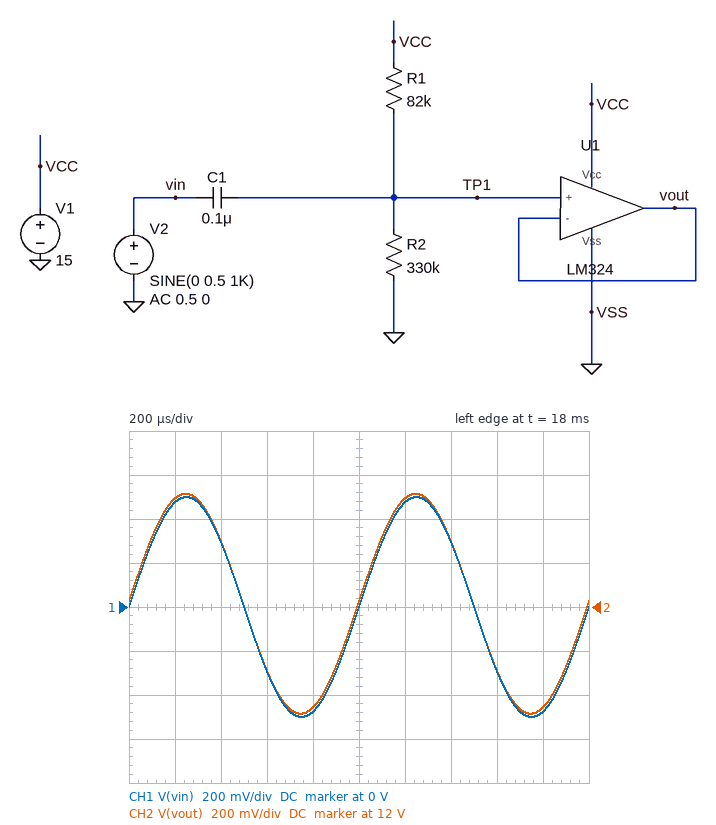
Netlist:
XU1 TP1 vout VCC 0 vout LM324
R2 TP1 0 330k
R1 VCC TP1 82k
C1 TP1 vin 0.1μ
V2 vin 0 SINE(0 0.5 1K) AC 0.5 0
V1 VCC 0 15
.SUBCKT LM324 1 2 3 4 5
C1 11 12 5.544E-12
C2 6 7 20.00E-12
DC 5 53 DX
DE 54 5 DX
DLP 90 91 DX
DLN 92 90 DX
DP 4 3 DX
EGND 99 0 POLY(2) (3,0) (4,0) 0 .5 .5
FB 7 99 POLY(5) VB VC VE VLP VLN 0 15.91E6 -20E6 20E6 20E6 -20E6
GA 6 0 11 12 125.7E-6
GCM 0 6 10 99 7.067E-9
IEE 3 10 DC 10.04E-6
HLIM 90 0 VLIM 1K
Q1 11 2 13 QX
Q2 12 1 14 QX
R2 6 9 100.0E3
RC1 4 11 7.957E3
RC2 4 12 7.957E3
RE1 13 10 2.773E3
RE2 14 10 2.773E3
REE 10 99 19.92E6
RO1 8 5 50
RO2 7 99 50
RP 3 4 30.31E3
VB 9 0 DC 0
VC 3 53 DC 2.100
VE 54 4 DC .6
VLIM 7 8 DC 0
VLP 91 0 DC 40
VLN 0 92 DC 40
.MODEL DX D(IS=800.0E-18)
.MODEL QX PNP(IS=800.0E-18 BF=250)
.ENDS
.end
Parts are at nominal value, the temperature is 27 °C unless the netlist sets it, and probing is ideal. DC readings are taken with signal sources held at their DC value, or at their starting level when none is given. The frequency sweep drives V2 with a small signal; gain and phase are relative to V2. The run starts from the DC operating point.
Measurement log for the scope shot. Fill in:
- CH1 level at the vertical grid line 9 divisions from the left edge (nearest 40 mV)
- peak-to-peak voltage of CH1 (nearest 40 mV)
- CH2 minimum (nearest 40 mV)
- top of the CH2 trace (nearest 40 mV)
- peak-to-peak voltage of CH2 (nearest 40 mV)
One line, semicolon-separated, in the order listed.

-480 mV; 1.00 V; 11.52 V; 12.52 V; 1.00 V
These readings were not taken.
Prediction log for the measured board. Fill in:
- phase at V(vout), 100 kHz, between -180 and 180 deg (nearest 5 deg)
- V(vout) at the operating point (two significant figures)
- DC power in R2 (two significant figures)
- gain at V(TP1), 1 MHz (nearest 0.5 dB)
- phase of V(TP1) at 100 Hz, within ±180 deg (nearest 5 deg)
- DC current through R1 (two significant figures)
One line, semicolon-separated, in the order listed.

-5 deg; 12 V; 440 µW; 0 dB; 15 deg; 36 µA
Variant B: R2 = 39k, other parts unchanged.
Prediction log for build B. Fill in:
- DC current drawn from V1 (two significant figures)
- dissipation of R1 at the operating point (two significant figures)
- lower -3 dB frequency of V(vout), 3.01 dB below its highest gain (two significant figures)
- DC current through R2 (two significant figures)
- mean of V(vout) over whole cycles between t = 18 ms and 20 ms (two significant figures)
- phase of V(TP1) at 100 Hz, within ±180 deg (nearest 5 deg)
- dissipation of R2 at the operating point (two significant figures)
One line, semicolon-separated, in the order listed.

630 µA; 1.3 mW; 61 Hz; 120 µA; 4.8 V; 30 deg; 600 µW
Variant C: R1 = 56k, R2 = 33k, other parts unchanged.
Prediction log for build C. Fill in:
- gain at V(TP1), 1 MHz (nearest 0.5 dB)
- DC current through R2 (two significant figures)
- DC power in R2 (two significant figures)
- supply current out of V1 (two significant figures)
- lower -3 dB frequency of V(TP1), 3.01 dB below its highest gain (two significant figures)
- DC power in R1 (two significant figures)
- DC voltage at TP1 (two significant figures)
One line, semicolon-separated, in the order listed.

0 dB; 170 µA; 940 µW; 670 µA; 77 Hz; 1.6 mW; 5.6 V
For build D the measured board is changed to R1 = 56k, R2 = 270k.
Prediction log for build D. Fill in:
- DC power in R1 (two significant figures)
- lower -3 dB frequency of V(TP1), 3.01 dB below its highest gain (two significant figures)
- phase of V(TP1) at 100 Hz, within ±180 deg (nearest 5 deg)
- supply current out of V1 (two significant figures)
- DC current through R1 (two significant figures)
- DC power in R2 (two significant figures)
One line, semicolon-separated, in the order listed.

120 µW; 34 Hz; 20 deg; 550 µA; 46 µA; 570 µW
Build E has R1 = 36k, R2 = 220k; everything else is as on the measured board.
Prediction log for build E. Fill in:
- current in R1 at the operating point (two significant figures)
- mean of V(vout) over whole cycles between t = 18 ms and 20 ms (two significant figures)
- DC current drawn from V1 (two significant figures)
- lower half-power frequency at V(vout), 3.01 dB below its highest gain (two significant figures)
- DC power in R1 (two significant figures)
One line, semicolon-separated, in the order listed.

59 µA; 13 V; 560 µA; 52 Hz; 120 µW
